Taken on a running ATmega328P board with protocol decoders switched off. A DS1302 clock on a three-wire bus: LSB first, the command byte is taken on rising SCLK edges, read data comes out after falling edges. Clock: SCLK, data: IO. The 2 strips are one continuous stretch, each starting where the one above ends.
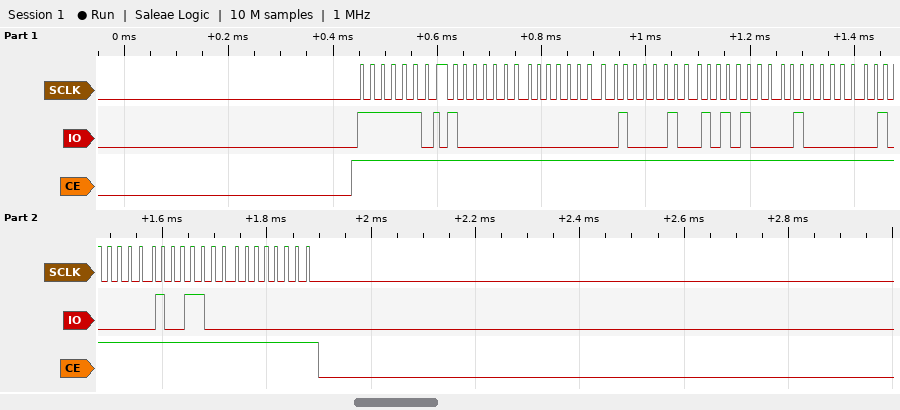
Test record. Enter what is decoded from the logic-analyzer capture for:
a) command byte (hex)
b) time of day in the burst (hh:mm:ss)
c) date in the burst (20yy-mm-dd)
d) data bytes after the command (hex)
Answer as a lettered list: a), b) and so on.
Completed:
a) 0xBF
b) 21:00:01
c) 2019-02-15
d) 01 00 21 15 02 02 19 00
